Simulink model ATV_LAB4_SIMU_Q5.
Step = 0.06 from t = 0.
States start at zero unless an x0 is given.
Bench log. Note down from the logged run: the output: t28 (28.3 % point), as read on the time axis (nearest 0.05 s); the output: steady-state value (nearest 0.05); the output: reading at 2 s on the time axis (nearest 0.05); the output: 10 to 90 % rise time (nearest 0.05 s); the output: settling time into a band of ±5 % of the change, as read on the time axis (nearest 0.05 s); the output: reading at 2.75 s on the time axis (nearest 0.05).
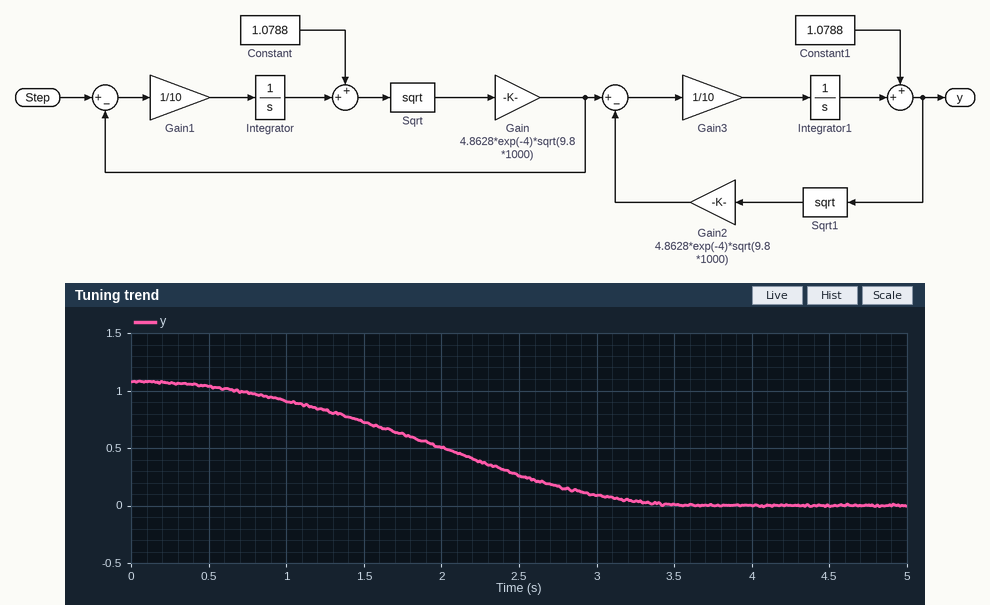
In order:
1.40 s
0.00
0.50
2.15 s
3.15 s
0.15
